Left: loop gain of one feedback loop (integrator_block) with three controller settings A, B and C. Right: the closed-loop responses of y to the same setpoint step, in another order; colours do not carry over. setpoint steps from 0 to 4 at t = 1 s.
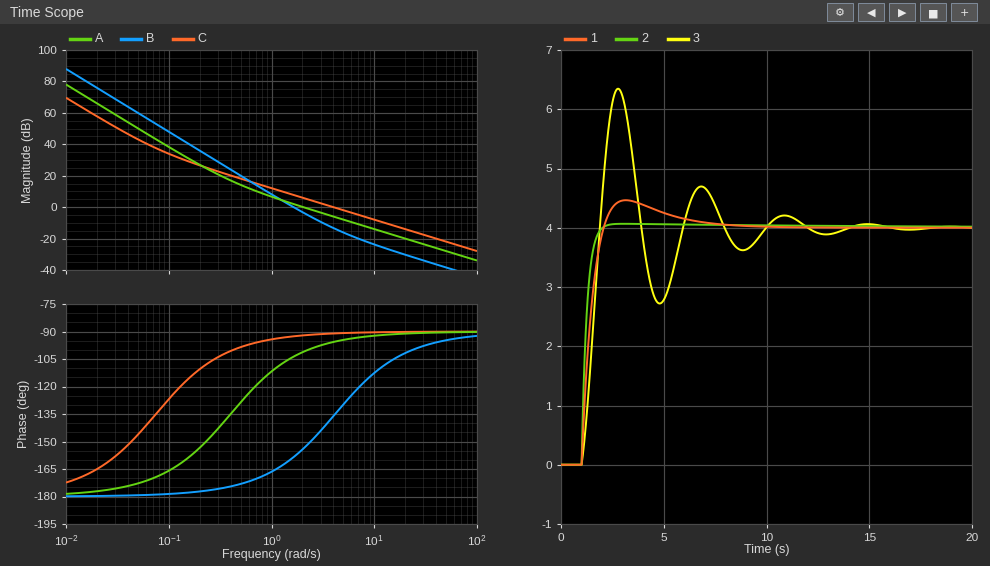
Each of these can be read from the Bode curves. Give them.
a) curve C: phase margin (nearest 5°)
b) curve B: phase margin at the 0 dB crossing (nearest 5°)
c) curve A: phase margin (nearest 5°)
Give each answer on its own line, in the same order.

90°
20°
80°
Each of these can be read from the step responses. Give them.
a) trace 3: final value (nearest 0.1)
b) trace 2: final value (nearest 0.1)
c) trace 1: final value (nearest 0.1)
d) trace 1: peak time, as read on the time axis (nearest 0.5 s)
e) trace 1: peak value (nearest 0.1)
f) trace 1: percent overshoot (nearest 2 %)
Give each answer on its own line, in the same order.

4.0
4.0
4.0
3.0 s
4.5
12 %
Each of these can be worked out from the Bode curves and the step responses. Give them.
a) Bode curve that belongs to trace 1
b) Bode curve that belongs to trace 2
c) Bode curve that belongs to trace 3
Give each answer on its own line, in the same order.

A
C
B
